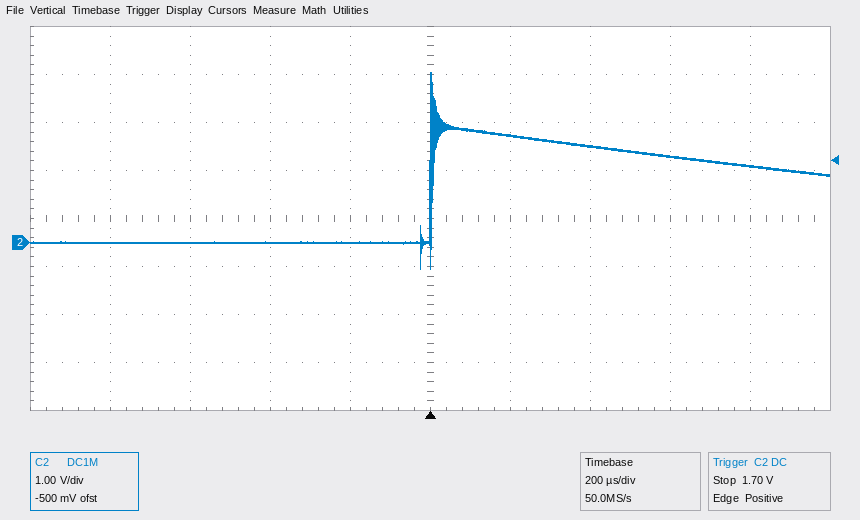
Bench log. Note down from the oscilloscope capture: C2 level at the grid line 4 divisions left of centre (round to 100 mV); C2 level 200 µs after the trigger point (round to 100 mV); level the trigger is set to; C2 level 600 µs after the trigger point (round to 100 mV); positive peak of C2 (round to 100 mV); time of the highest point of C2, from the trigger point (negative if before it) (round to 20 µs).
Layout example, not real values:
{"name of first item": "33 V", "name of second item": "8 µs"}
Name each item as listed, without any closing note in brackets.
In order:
{"C2 level at the grid line 4 divisions left of centre": "0.0 V", "C2 level 200 µs after the trigger point": "2.2 V", "level the trigger is set to": "1.70 V", "C2 level 600 µs after the trigger point": "1.8 V", "positive peak of C2": "3.5 V", "time of the highest point of C2, from the trigger point (negative if before it)": "0 µs"}
